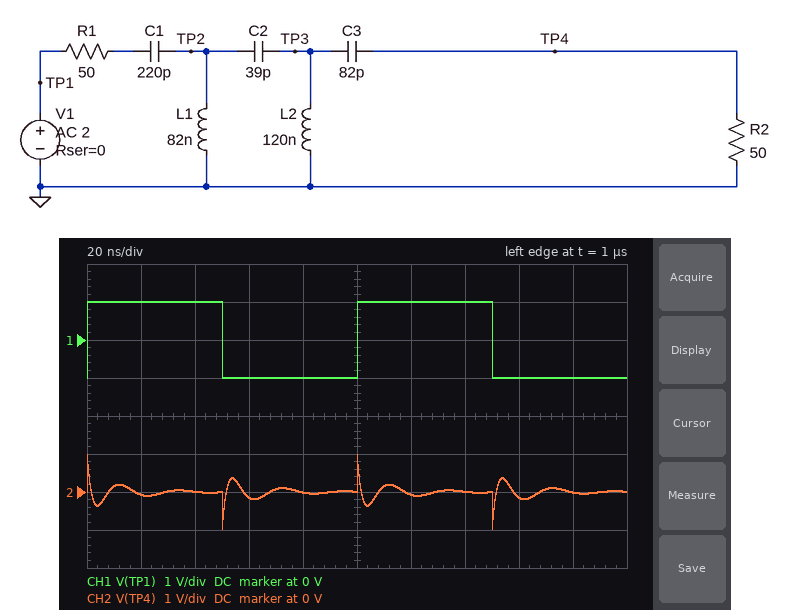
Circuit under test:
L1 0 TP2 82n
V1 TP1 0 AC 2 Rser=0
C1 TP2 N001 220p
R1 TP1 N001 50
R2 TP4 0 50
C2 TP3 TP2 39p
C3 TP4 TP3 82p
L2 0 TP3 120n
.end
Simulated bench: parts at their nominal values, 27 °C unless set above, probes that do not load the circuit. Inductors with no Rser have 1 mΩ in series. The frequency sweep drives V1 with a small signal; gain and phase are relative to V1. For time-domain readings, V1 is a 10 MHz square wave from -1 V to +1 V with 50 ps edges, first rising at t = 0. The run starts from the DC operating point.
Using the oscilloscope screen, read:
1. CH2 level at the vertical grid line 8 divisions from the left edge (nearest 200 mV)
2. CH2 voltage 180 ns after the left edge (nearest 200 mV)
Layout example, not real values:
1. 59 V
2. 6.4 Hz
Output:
1. -200 mV
2. 0 V
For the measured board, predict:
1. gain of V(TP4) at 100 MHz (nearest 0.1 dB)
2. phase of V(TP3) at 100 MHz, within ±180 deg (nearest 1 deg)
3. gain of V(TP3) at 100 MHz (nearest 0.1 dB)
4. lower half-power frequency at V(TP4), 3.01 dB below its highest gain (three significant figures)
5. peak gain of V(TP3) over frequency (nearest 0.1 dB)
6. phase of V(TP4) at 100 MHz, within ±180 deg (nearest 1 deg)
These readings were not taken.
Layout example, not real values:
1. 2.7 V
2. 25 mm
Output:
1. -6.3 dB
2. 67 deg
3. -5.7 dB
4. 45.7 MHz
5. -5.3 dB
6. 88 deg
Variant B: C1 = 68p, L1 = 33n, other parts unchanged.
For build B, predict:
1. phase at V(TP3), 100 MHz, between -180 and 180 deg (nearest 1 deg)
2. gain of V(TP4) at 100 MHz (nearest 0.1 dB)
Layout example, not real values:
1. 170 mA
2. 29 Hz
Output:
1. 114 deg
2. -9.1 dB
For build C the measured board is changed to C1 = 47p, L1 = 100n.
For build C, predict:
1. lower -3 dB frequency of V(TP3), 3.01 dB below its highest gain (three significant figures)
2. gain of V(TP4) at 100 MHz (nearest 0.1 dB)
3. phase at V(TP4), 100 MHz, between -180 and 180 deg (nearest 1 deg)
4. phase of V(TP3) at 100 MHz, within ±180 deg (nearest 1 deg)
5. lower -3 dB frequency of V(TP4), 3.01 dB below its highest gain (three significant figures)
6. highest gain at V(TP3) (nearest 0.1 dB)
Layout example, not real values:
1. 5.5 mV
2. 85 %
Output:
1. 42.2 MHz
2. -6.1 dB
3. 98 deg
4. 77 deg
5. 43.6 MHz
6. -4.6 dB
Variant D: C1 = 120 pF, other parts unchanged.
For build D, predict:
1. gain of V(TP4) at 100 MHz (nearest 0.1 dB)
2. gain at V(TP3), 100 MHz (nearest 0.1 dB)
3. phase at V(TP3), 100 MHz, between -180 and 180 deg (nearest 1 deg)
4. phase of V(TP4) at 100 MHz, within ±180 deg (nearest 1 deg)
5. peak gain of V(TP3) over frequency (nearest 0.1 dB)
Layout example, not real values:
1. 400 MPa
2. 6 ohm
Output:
1. -6.2 dB
2. -5.6 dB
3. 70 deg
4. 92 deg
5. -5.0 dB
